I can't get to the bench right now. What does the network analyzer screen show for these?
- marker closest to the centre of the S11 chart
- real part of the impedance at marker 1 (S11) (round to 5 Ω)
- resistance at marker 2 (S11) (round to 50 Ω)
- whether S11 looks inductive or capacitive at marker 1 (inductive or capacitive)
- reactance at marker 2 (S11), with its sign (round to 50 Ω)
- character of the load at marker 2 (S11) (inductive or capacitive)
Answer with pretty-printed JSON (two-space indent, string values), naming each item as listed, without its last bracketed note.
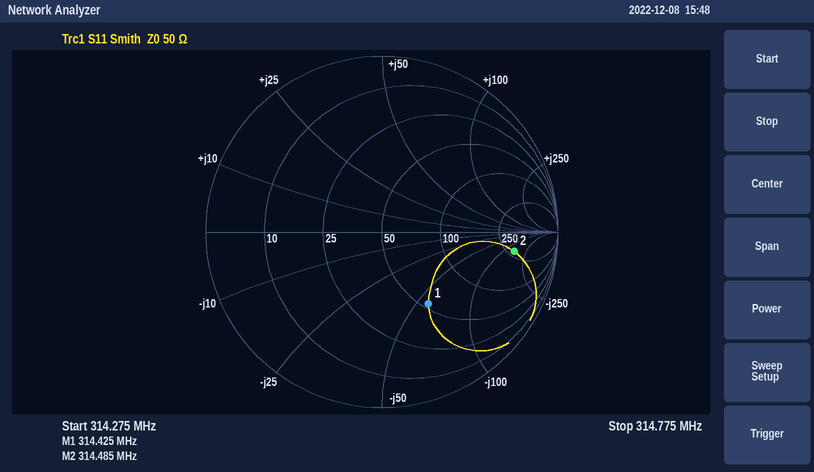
{
  "marker closest to the centre of the S11 chart": "marker 1",
  "real part of the impedance at marker 1 (S11)": "55 Ω",
  "resistance at marker 2 (S11)": "300 Ω",
  "whether S11 looks inductive or capacitive at marker 1": "capacitive",
  "reactance at marker 2 (S11), with its sign": "-150 Ω",
  "character of the load at marker 2 (S11)": "capacitive"
}
